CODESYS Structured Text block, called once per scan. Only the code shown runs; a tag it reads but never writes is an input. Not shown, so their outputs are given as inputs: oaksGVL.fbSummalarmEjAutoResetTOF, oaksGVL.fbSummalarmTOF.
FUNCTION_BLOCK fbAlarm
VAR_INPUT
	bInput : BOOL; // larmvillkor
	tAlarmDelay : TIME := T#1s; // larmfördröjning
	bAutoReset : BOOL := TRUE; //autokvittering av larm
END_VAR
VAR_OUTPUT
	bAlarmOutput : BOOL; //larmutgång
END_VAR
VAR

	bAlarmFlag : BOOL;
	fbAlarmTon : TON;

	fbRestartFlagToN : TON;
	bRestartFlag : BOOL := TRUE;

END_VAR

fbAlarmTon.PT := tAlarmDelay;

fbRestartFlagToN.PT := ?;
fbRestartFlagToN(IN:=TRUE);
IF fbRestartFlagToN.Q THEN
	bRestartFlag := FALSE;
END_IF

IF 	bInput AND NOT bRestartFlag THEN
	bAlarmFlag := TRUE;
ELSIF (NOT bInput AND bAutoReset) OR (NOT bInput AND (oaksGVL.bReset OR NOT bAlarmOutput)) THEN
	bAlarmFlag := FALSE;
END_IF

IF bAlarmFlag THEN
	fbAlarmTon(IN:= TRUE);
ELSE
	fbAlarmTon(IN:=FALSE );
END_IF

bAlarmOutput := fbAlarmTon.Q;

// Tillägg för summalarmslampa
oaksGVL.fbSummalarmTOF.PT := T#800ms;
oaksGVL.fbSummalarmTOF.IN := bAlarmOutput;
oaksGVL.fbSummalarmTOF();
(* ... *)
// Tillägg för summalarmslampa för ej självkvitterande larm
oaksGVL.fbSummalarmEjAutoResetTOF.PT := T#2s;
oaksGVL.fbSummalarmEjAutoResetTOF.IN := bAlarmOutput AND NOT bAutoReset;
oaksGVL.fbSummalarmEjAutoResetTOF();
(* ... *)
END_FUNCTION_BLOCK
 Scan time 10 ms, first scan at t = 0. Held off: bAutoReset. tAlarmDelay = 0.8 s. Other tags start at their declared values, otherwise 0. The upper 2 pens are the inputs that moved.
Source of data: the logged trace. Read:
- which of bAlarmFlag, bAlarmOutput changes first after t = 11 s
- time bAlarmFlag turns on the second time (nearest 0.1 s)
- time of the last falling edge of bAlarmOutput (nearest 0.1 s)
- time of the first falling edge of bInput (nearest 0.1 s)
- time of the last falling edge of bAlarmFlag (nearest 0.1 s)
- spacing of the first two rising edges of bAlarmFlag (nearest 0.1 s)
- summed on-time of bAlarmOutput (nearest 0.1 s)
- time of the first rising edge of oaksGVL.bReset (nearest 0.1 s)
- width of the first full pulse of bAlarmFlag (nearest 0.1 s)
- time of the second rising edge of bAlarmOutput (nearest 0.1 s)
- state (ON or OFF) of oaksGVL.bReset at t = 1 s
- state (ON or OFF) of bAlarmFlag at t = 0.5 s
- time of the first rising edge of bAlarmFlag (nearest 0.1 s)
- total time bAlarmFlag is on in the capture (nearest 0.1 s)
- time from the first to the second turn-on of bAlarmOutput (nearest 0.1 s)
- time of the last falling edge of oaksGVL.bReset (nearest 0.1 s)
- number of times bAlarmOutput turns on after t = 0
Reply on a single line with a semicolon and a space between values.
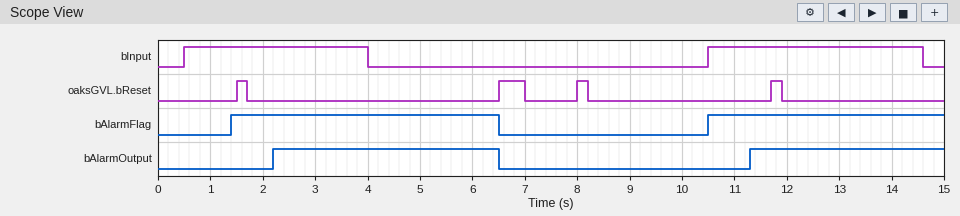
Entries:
bAlarmOutput; 10.5 s; 6.5 s; 4.0 s; 6.5 s; 9.1 s; 8.0 s; 1.5 s; 5.1 s; 11.3 s; OFF; OFF; 1.4 s; 9.6 s; 9.1 s; 11.9 s; 2
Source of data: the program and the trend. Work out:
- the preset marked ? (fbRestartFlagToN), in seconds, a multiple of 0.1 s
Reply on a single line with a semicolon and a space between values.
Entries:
1.4 s
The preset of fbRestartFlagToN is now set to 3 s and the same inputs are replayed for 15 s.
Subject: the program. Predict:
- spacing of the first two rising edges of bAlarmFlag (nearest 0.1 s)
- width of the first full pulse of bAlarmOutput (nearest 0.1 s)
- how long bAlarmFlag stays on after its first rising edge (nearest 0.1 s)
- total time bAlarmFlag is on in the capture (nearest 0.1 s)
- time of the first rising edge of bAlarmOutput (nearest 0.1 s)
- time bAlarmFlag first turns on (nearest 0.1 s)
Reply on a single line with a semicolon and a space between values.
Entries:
7.5 s; 2.7 s; 3.5 s; 8.0 s; 3.8 s; 3.0 s
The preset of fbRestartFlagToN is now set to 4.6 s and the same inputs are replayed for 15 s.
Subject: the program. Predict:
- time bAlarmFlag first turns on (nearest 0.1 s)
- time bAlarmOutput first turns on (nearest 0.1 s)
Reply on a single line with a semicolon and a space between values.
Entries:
10.5 s; 11.3 s
